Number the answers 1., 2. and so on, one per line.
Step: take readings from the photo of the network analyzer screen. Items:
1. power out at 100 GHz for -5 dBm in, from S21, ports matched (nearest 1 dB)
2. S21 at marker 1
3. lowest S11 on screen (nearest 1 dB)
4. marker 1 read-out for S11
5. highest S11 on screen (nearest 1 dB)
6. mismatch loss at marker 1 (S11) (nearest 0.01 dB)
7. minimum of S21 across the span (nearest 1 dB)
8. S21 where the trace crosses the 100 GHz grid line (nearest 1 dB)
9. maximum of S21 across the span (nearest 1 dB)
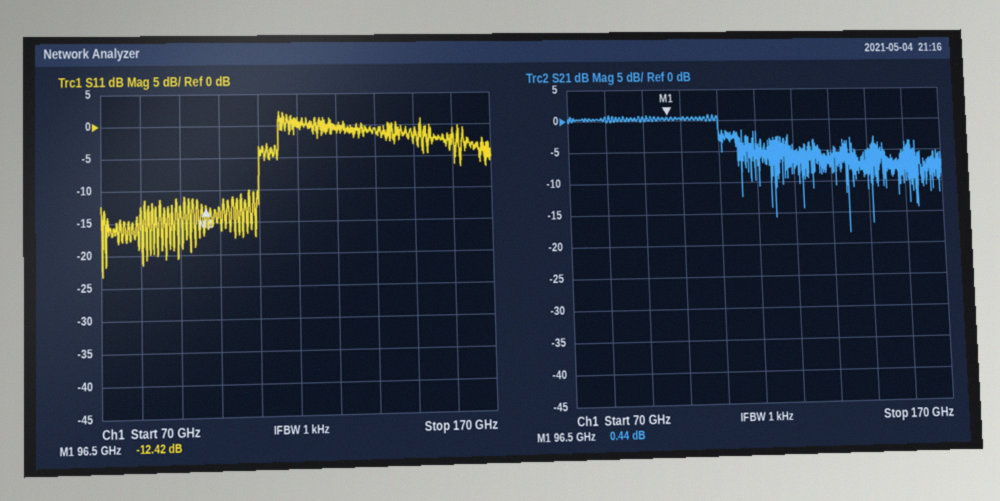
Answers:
1. -5 dBm
2. 0.44 dB
3. -23 dB
4. -12.42 dB
5. 2 dB
6. 0.26 dB
7. -18 dB
8. 0 dB
9. 1 dB
